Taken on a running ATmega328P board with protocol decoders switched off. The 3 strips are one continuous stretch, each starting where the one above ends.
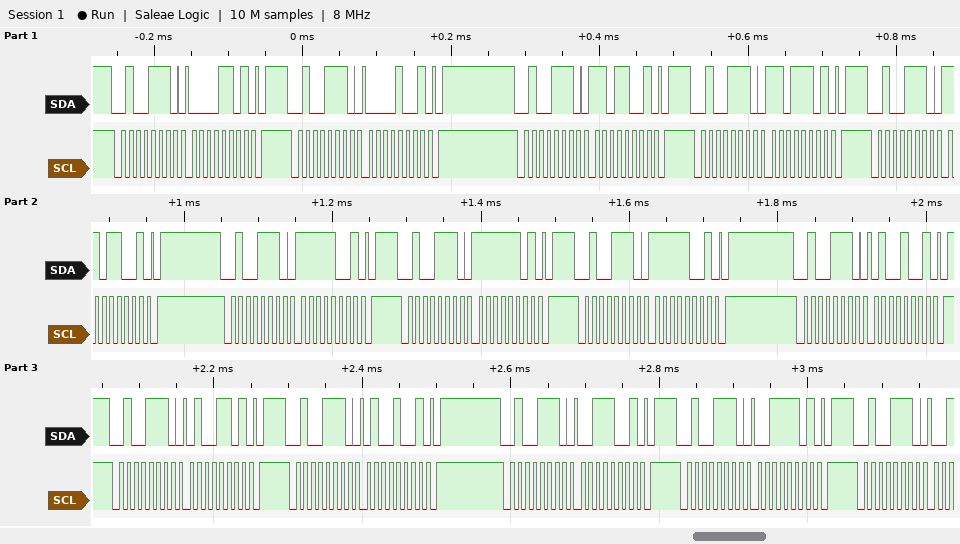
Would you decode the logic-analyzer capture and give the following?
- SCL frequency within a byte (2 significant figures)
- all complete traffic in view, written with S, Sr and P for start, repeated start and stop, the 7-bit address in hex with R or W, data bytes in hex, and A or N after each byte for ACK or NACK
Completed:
100 kHz
S 27W A 0D A P S 27W A 09 A P S 27W A D9 A P S 27W A DD A P S 27W A D9 A P S 27W A F9 A P S 27W A FD A P S 27W A F9 A P S 27W A 49 A P S 27W A 4D A P S 27W A 49 A P S 27W A 39 A P S 27W A 3D A P S 27W A
